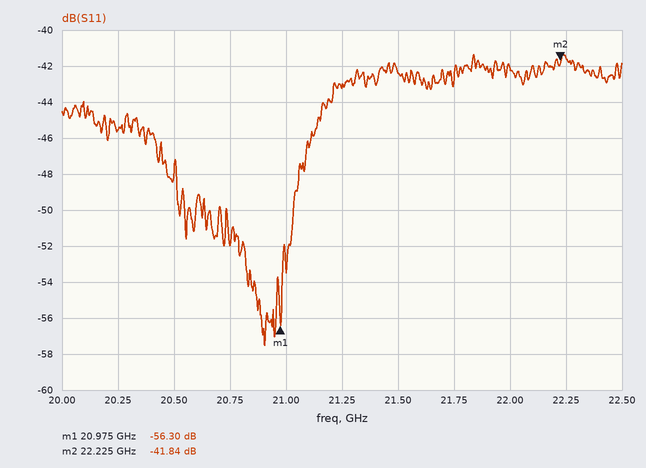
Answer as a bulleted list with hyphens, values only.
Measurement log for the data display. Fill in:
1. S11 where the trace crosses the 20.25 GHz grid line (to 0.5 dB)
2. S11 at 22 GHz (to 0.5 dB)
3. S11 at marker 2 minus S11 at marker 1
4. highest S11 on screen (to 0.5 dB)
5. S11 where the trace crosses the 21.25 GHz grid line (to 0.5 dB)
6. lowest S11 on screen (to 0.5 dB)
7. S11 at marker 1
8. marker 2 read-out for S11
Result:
- -45.5 dB
- -42.0 dB
- 14.46 dB
- -41.5 dB
- -43.0 dB
- -57.5 dB
- -56.30 dB
- -41.84 dB
